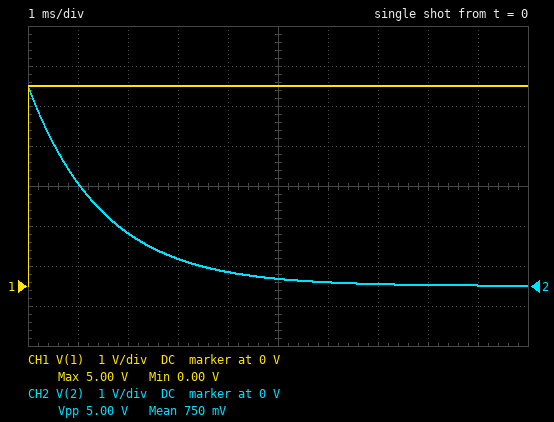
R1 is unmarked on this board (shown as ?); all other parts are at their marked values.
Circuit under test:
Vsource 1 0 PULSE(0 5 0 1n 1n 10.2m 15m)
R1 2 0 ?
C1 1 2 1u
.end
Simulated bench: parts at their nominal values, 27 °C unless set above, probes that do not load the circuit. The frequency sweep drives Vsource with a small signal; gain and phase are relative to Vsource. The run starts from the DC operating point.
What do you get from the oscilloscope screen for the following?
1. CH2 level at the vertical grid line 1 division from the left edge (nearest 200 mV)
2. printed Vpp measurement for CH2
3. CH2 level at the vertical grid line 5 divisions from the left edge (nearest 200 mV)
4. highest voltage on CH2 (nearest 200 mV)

2.6 V
5.00 V
200 mV
5.0 V
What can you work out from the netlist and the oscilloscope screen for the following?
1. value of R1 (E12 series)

1.5 kΩ
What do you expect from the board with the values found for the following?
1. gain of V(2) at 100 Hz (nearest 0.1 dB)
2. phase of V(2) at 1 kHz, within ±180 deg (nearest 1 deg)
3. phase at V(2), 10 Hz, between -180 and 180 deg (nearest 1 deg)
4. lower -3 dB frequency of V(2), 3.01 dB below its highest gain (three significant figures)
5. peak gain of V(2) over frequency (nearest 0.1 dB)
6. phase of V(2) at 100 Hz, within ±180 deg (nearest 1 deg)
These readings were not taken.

-3.3 dB
6 deg
85 deg
106 Hz
0 dB
47 deg
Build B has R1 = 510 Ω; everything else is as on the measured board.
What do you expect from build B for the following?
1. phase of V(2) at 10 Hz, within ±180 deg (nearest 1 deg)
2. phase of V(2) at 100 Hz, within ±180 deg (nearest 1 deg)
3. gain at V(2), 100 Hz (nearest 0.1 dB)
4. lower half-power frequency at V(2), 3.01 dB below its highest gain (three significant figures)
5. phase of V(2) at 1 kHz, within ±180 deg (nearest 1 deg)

88 deg
72 deg
-10.3 dB
312 Hz
17 deg
